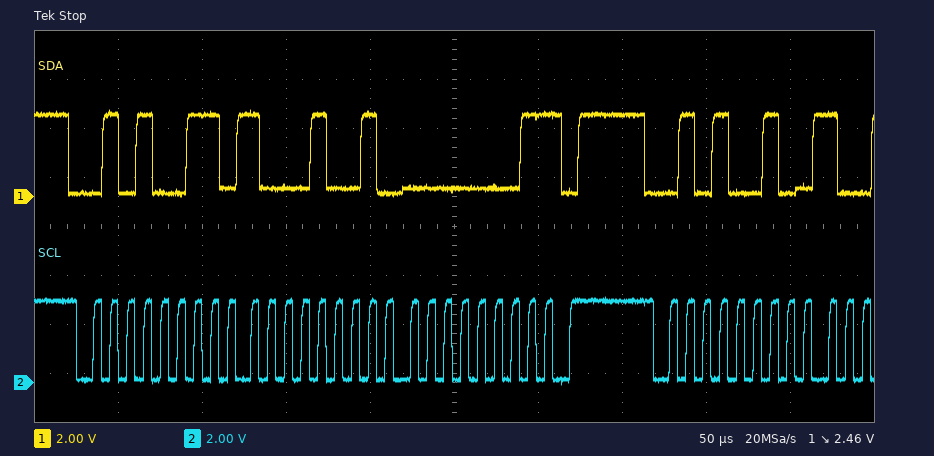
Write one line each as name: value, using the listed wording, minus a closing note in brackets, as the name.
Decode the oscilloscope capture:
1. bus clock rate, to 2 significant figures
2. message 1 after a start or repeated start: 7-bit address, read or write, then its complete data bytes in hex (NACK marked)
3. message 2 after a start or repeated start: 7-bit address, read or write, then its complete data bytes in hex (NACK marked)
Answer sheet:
bus clock rate, to 2 significant figures: 100 kHz
message 1 after a start or repeated start: 7-bit address, read or write, then its complete data bytes in hex: 0x29 read: 89 01 NACK
message 2 after a start or repeated start: 7-bit address, read or write, then its complete data bytes in hex: 0x29 write
